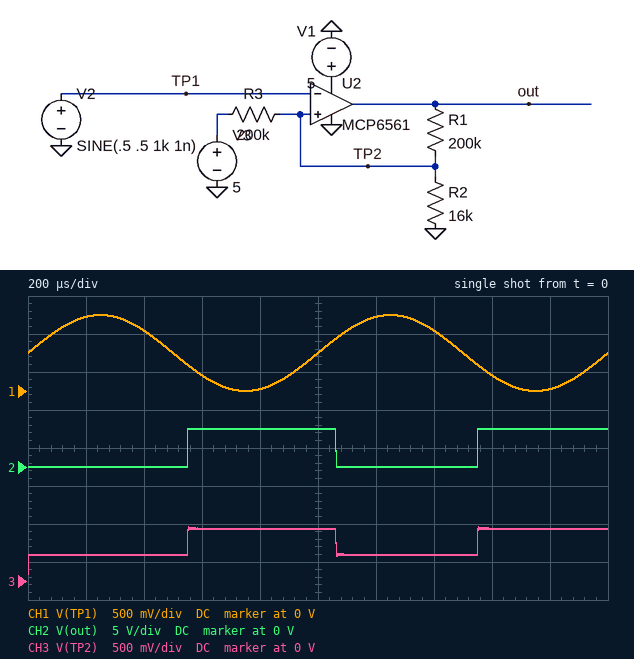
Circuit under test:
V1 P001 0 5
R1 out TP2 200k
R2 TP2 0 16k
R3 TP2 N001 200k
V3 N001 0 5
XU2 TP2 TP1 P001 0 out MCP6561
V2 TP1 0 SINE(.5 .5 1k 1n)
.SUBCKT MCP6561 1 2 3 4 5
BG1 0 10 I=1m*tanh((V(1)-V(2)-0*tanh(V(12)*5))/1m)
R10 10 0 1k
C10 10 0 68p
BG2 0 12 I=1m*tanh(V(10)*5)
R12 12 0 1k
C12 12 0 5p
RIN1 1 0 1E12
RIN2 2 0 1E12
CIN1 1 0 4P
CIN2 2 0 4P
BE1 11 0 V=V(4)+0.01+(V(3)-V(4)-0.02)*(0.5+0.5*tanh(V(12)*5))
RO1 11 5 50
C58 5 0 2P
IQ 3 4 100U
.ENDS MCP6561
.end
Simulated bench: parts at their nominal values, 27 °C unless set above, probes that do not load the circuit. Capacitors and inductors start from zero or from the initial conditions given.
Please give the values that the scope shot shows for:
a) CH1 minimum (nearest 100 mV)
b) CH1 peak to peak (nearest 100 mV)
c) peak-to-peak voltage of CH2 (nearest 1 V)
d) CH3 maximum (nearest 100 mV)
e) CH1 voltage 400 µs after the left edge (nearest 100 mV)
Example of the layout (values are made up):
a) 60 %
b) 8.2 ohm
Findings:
a) 0 V
b) 1.0 V
c) 5 V
d) 700 mV
e) 800 mV
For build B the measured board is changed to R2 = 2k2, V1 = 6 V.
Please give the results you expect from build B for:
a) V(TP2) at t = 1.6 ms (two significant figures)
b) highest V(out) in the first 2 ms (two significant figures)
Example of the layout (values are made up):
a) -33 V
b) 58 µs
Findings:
a) 54 mV
b) 6.0 V
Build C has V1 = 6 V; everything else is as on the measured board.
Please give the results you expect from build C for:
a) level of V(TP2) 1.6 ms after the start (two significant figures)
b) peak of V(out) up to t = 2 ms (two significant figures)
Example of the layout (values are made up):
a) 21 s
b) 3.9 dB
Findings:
a) 760 mV
b) 6.0 V
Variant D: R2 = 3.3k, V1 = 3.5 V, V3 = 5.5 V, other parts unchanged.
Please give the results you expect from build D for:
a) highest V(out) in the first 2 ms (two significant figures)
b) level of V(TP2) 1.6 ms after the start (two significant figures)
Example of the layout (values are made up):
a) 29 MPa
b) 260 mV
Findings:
a) 3.5 V
b) 88 mV
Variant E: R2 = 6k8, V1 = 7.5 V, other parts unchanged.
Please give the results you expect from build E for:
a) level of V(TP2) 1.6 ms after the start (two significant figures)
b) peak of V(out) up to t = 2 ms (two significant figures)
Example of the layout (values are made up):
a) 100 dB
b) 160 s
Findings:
a) 160 mV
b) 7.5 V
